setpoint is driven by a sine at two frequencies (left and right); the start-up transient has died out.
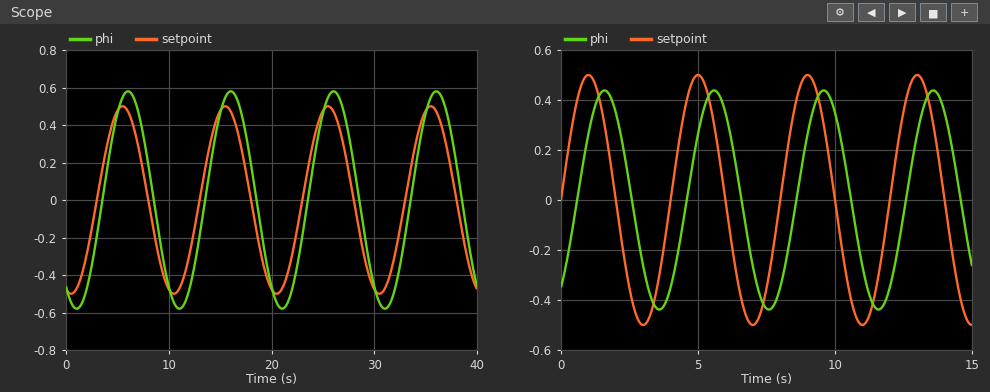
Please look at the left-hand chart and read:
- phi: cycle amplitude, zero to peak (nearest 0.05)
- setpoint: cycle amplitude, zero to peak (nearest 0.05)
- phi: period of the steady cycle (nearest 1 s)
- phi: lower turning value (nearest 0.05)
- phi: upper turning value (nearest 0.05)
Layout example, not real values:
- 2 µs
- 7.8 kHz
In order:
- 0.60
- 0.50
- 10 s
- -0.60
- 0.60
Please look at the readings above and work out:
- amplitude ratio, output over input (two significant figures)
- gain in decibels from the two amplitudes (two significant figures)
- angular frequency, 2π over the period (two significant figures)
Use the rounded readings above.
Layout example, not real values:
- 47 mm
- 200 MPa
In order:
- 1.2
- 1.6 dB
- 0.63 rad/s
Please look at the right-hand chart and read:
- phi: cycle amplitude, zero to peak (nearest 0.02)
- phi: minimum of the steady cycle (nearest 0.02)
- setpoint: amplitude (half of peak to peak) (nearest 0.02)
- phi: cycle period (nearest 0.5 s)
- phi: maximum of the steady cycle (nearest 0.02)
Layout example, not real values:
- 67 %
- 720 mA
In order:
- 0.44
- -0.44
- 0.50
- 4.0 s
- 0.44
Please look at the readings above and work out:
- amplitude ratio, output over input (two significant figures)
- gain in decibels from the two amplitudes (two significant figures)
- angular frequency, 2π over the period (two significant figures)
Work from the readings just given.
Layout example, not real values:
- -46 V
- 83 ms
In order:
- 0.88
- -1.1 dB
- 1.6 rad/s
